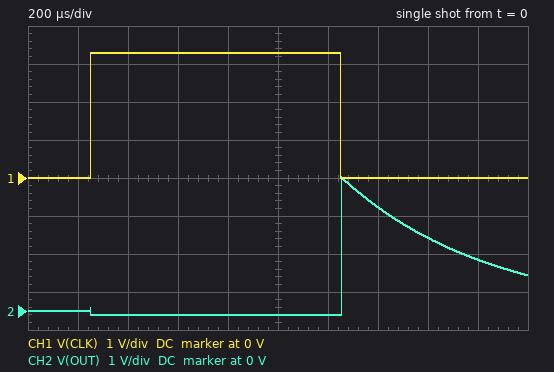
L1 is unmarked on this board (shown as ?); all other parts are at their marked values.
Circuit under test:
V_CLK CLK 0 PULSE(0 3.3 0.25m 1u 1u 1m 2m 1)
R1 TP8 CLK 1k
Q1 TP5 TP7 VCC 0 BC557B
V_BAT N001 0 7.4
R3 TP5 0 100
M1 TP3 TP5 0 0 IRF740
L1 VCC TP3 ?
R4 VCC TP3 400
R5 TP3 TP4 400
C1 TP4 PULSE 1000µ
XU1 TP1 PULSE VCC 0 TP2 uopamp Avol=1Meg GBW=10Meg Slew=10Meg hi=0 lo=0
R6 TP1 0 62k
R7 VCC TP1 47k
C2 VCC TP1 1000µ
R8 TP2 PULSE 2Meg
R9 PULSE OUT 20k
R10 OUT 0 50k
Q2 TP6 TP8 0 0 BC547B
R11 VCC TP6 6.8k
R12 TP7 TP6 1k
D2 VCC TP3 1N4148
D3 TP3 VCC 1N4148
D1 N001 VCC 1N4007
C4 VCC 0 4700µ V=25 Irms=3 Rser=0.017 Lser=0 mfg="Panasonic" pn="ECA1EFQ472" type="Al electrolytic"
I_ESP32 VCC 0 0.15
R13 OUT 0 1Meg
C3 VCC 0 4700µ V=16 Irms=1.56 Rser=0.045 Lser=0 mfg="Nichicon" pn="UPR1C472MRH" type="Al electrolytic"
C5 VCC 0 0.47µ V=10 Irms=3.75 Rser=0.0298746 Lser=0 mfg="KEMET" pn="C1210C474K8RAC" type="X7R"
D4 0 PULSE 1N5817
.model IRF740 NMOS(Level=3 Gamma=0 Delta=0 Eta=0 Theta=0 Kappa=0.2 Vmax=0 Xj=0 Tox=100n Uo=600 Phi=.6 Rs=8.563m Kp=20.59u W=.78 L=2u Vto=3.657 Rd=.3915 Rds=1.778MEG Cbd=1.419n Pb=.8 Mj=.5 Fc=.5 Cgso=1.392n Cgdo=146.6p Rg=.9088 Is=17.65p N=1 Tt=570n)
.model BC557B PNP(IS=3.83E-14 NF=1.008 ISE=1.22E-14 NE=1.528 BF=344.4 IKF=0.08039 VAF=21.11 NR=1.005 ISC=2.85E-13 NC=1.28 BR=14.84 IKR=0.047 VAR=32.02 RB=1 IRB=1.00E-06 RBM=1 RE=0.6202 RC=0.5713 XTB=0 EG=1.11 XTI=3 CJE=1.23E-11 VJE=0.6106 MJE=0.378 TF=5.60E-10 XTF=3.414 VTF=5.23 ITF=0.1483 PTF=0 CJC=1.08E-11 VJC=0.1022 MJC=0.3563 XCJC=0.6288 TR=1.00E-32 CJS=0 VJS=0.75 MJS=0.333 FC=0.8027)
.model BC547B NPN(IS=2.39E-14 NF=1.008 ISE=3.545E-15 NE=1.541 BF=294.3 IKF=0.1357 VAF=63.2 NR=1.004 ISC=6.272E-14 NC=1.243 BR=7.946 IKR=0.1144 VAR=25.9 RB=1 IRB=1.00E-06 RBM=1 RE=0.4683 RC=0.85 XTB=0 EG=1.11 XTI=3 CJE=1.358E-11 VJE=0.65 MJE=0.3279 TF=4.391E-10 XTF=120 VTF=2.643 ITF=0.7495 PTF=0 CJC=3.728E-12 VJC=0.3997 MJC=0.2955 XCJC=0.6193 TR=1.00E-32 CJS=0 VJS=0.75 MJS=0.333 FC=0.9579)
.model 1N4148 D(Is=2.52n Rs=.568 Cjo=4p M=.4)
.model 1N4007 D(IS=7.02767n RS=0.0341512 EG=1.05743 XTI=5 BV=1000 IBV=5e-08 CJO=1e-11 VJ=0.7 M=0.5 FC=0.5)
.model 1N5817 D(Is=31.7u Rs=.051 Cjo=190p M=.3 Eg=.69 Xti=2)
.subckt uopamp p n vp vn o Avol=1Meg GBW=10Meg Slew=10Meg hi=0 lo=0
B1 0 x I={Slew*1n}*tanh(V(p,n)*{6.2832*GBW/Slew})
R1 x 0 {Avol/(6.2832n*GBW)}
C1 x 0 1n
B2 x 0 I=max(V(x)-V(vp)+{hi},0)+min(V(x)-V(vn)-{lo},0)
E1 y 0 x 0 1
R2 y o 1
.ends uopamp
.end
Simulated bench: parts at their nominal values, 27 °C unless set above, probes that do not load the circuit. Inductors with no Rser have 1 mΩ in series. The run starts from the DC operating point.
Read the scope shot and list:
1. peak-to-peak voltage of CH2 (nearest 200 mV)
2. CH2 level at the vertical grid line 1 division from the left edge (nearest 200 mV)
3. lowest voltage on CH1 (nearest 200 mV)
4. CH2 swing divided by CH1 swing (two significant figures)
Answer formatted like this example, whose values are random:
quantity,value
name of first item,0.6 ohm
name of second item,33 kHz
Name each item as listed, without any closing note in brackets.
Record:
quantity,value
peak-to-peak voltage of CH2,3.6 V
CH2 level at the vertical grid line 1 division from the left edge,0 V
lowest voltage on CH1,0 V
CH2 swing divided by CH1 swing,1.1
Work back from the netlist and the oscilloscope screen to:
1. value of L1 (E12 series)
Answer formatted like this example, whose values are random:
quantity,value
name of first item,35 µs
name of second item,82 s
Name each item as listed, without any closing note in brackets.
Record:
quantity,value
value of L1,330 µH
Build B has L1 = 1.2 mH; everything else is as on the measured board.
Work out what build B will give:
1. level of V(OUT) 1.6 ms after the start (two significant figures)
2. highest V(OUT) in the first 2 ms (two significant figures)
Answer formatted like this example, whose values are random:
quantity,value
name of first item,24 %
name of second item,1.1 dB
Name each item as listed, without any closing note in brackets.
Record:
quantity,value
level of V(OUT) 1.6 ms after the start,1.2 V
highest V(OUT) in the first 2 ms,1.4 V
